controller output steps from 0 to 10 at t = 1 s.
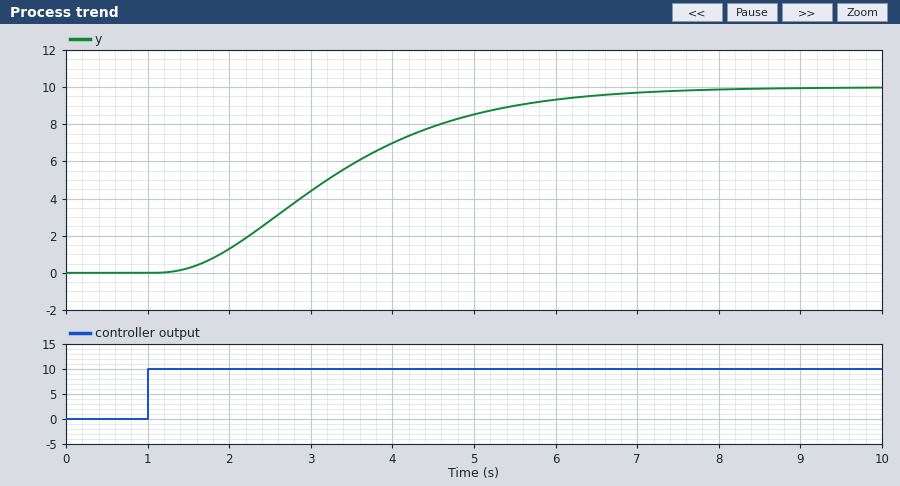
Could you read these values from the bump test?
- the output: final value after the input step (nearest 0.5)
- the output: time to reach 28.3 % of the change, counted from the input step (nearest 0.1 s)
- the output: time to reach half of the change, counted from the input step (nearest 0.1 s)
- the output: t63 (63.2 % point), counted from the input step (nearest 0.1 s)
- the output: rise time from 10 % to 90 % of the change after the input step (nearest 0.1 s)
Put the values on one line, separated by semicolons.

10.0; 1.5 s; 2.2 s; 2.7 s; 3.6 s
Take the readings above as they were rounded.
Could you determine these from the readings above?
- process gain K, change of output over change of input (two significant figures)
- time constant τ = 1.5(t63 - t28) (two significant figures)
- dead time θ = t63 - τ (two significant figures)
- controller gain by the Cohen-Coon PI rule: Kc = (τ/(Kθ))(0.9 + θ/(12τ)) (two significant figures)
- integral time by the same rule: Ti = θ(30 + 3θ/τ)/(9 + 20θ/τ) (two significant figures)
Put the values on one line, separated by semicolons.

1.0; 1.8 s; 0.90 s; 1.9; 1.5 s
